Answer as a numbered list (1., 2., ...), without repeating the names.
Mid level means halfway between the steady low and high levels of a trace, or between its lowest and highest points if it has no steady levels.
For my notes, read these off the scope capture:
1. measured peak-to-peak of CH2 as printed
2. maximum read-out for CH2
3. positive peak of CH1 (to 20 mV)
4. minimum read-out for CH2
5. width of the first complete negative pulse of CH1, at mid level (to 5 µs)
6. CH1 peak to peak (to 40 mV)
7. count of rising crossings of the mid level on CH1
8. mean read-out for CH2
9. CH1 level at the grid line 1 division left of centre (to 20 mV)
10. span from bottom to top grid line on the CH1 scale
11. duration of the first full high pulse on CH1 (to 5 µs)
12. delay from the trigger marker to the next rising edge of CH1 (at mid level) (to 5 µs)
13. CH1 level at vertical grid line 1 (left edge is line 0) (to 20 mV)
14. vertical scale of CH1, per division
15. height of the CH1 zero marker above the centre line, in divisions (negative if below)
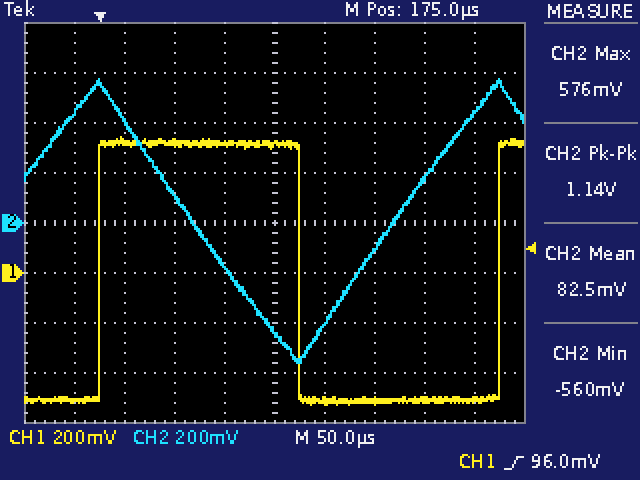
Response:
1. 1.14 V
2. 576 mV
3. 540 mV
4. -560 mV
5. 200 µs
6. 1.08 V
7. 2
8. 82.5 mV
9. 520 mV
10. 1.6 V
11. 200 µs
12. 400 µs
13. -520 mV
14. 200 mV
15. -1.0 div
